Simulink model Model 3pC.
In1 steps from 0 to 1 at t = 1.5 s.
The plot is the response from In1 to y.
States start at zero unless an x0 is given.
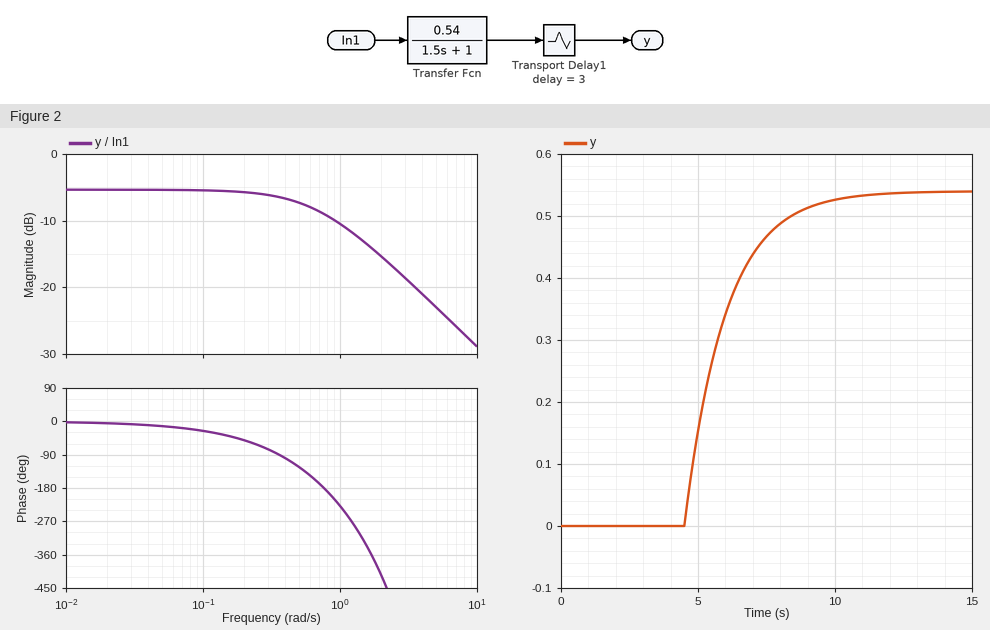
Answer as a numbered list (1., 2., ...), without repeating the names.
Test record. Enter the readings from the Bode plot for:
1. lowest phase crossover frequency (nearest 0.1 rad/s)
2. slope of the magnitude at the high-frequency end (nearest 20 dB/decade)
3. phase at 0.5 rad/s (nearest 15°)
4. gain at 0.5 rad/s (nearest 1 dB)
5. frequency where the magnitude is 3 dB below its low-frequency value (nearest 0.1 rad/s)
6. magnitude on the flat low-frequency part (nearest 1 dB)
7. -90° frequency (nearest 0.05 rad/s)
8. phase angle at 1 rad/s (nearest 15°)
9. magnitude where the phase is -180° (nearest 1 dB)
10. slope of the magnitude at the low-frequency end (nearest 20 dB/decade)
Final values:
1. 0.8 rad/s
2. -20 dB/decade
3. -120°
4. -7 dB
5. 0.7 rad/s
6. -5 dB
7. 0.35 rad/s
8. -225°
9. -9 dB
10. 0 dB/decade
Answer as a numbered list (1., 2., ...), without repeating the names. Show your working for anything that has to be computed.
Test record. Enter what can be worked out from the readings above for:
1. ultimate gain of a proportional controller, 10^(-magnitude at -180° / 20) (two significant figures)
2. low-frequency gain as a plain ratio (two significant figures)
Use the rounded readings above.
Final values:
1. 10^(9 / 20) = 2.8
2. 10^(-5 / 20) = 0.56
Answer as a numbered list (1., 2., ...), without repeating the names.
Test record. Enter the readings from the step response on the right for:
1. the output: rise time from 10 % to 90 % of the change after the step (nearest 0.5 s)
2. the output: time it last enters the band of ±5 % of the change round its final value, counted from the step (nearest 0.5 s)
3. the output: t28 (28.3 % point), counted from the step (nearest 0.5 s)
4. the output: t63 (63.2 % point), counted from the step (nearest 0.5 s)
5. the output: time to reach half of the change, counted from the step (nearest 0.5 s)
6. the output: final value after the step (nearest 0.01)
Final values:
1. 3.5 s
2. 7.5 s
3. 3.5 s
4. 4.5 s
5. 4.0 s
6. 0.54
